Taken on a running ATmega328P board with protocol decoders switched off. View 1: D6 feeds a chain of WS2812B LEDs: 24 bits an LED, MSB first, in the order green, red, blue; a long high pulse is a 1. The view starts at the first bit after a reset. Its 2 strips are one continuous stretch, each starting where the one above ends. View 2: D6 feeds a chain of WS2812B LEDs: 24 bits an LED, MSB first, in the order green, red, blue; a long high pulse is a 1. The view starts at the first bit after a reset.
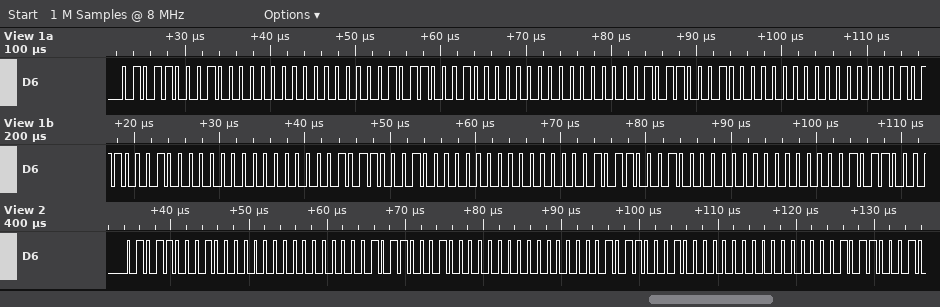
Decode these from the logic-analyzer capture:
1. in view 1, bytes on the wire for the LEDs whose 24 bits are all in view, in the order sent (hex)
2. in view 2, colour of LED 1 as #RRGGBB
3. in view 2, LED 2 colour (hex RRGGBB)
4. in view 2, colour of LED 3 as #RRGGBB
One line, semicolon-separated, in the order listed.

58 80 00 58 80 00 58 80 00 58 80 00 58 80 00 58 80 00; #805800; #805800; #805800
